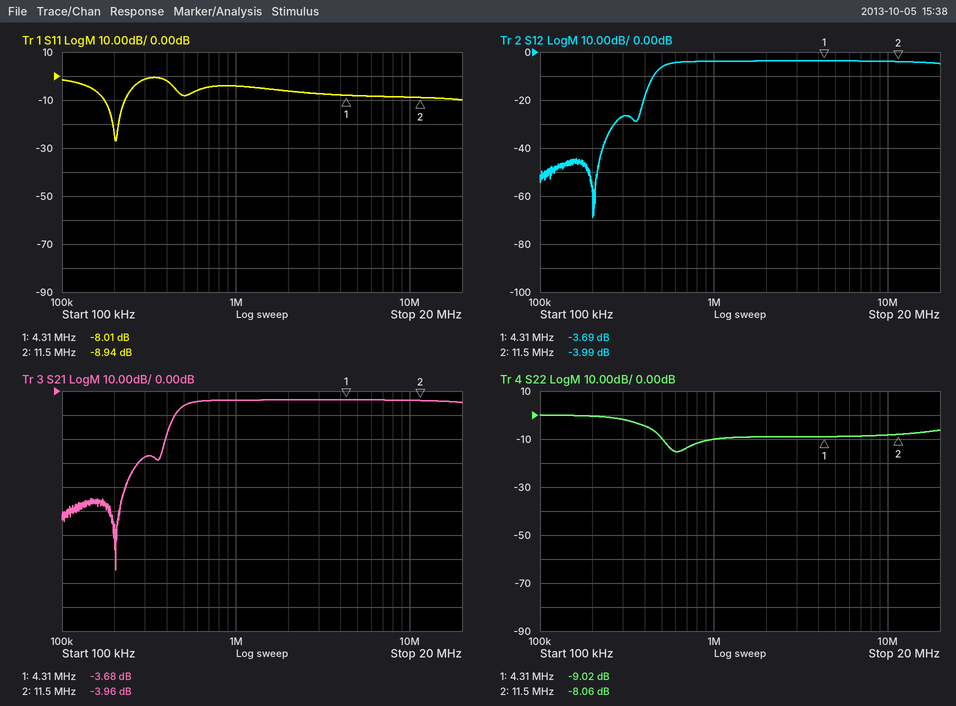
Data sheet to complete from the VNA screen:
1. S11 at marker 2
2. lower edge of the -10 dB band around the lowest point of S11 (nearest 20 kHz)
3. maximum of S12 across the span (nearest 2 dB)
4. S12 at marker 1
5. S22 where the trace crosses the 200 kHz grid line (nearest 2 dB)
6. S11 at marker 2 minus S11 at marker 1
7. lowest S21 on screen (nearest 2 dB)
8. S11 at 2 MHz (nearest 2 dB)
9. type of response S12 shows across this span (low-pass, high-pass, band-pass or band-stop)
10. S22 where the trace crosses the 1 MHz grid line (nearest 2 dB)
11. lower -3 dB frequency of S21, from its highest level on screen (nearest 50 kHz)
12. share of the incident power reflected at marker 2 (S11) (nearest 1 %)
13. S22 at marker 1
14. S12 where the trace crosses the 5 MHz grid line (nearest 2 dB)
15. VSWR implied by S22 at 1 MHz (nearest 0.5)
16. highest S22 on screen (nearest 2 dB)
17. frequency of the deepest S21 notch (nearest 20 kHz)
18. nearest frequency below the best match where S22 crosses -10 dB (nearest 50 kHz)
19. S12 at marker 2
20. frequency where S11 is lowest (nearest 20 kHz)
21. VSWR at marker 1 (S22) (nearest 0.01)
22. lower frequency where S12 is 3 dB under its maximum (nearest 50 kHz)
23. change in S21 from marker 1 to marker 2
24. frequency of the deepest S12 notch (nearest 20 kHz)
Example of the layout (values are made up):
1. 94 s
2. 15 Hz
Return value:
1. -8.94 dB
2. 180 kHz
3. -4 dB
4. -3.69 dB
5. 0 dB
6. -0.93 dB
7. -74 dB
8. -6 dB
9. high-pass
10. -10 dB
11. 500 kHz
12. 13 %
13. -9.02 dB
14. -4 dB
15. 2.0
16. 0 dB
17. 200 kHz
18. 500 kHz
19. -3.99 dB
20. 200 kHz
21. 2.10
22. 500 kHz
23. -0.28 dB
24. 200 kHz
